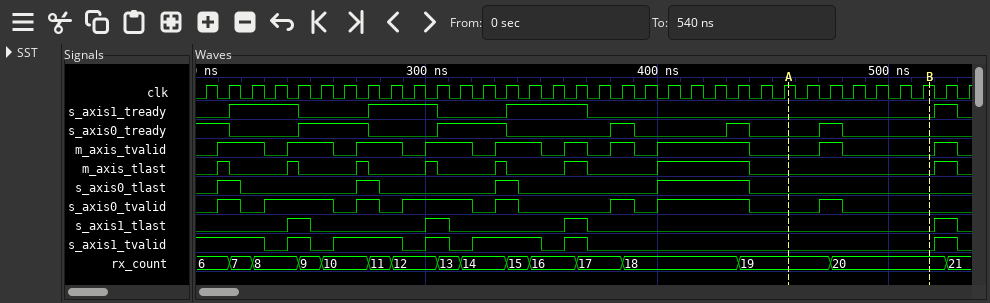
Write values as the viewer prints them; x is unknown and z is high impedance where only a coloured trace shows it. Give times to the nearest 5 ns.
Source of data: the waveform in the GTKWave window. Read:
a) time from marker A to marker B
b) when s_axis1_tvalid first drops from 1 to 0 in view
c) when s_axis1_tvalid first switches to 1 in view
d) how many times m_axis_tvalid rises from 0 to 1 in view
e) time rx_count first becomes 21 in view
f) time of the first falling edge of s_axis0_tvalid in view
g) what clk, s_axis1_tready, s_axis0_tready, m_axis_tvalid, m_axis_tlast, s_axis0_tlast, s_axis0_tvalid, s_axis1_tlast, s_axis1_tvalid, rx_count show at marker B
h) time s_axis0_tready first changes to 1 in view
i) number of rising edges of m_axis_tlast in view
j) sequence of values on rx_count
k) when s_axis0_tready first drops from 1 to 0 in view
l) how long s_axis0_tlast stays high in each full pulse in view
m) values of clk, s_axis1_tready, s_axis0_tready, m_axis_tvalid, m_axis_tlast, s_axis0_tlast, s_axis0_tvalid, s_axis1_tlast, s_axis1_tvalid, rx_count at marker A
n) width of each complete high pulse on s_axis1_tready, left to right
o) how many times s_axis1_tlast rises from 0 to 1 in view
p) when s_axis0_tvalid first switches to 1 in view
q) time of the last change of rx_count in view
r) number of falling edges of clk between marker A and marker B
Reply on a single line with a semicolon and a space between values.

60 ns; 230 ns; 240 ns; 10; 525 ns; 220 ns; clk=1, s_axis1_tready=0, s_axis0_tready=0, m_axis_tvalid=0, m_axis_tlast=0, s_axis0_tlast=0, s_axis0_tvalid=0, s_axis1_tlast=0, s_axis1_tvalid=0, rx_count=20; 245 ns; 8; 6, 7, 8, 9, 10, 11, 12, 13, 14, 15, 16, 17, 18, 19, 20, 21; 215 ns; 10 ns, 10 ns, 10 ns, 40 ns; clk=1, s_axis1_tready=0, s_axis0_tready=0, m_axis_tvalid=0, m_axis_tlast=0, s_axis0_tlast=0, s_axis0_tvalid=0, s_axis1_tlast=0, s_axis1_tvalid=0, rx_count=19; 30 ns, 30 ns, 35 ns, 10 ns; 4; 210 ns; 525 ns; 6
